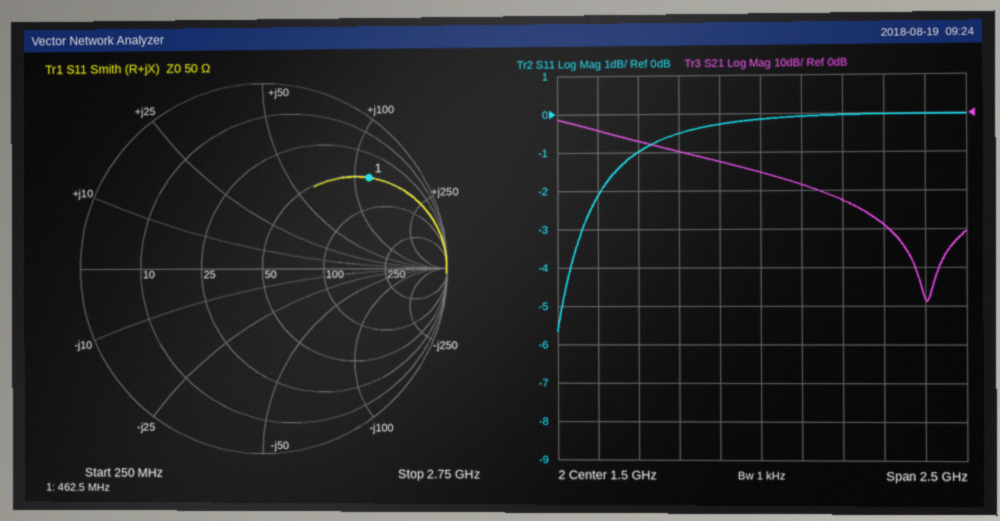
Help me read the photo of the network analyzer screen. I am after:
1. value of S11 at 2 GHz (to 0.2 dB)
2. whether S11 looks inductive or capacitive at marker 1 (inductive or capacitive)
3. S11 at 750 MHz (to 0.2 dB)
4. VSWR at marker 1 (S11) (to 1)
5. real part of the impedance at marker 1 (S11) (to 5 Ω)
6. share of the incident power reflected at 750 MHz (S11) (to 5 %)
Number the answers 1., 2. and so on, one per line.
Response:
1. 0.0 dB
2. inductive
3. -1.0 dB
4. 7
5. 50 Ω
6. 80 %
